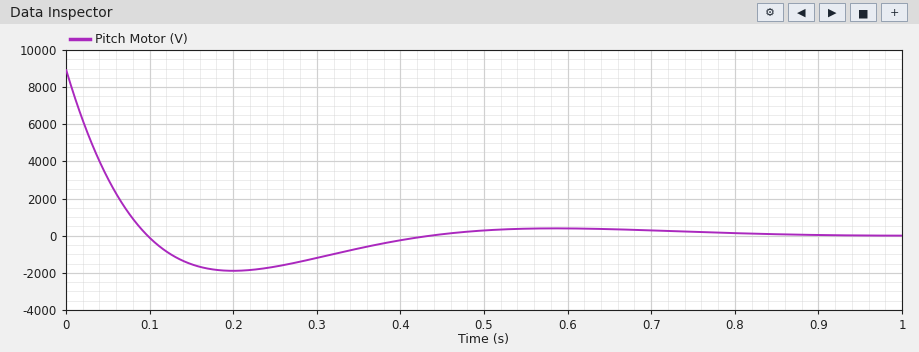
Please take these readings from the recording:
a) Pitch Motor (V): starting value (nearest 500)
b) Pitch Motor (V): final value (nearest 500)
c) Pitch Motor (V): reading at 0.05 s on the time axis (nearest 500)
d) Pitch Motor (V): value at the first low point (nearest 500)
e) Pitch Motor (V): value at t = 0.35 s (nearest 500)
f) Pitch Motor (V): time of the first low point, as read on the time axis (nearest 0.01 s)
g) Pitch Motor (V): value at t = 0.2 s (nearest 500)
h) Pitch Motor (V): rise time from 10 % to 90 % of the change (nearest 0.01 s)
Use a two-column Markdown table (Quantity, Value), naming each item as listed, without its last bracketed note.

| Quantity | Value |
|---|---|
| Pitch Motor (V): starting value | 9000 |
| Pitch Motor (V): final value | 0 |
| Pitch Motor (V): reading at 0.05 s on the time axis | 3000 |
| Pitch Motor (V): value at the first low point | -2000 |
| Pitch Motor (V): value at t = 0.35 s | -500 |
| Pitch Motor (V): time of the first low point, as read on the time axis | 0.20 s |
| Pitch Motor (V): value at t = 0.2 s | -2000 |
| Pitch Motor (V): rise time from 10 % to 90 % of the change | 0.07 s |
